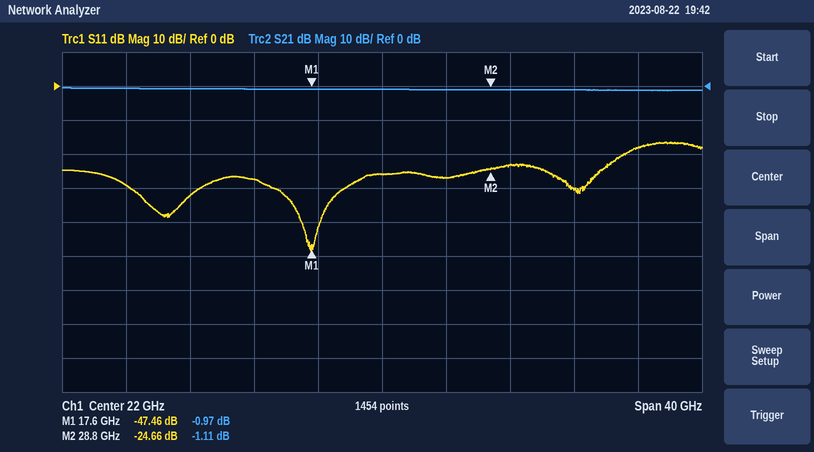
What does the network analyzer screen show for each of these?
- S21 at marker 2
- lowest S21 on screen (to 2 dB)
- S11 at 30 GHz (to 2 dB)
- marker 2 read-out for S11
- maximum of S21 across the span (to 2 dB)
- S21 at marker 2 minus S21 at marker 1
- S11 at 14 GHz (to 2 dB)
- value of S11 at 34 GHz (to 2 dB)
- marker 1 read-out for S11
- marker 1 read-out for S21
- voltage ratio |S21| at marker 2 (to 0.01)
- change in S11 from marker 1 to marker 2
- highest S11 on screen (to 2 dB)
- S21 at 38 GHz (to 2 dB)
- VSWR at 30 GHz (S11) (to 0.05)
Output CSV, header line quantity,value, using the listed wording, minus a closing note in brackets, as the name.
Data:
quantity,value
S21 at marker 2,-1.11 dB
lowest S21 on screen,-2 dB
S11 at 30 GHz,-24 dB
marker 2 read-out for S11,-24.66 dB
maximum of S21 across the span,0 dB
S21 at marker 2 minus S21 at marker 1,-0.14 dB
S11 at 14 GHz,-28 dB
value of S11 at 34 GHz,-30 dB
marker 1 read-out for S11,-47.46 dB
marker 1 read-out for S21,-0.97 dB
voltage ratio |S21| at marker 2,0.88
change in S11 from marker 1 to marker 2,22.80 dB
highest S11 on screen,-16 dB
S21 at 38 GHz,-2 dB
VSWR at 30 GHz (S11),1.15
